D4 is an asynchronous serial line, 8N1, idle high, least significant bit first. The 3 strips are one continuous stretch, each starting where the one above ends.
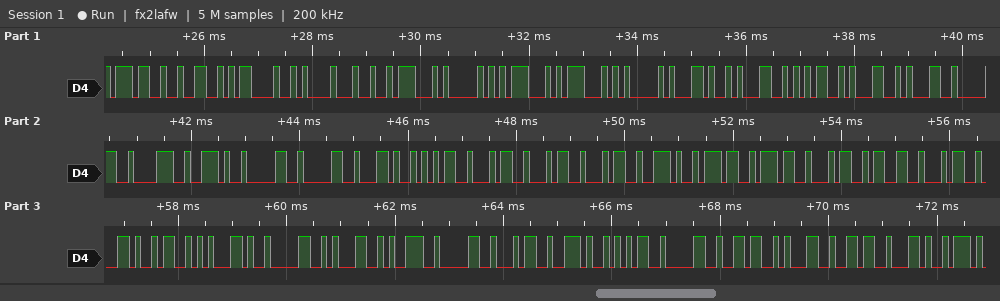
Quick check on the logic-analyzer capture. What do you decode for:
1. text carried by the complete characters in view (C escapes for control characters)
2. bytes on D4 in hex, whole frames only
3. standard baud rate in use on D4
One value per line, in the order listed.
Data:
"72\r\n$GPGGA,151108.00,5444.77434,S,01904.50616,"
37 32 0D 0A 24 47 50 47 47 41 2C 31 35 31 31 30 38 2E 30 30 2C 35 34 34 34 2E 37 37 34 33 34 2C 53 2C 30 31 39 30 34 2E 35 30 36 31 36 2C
9600 baud
